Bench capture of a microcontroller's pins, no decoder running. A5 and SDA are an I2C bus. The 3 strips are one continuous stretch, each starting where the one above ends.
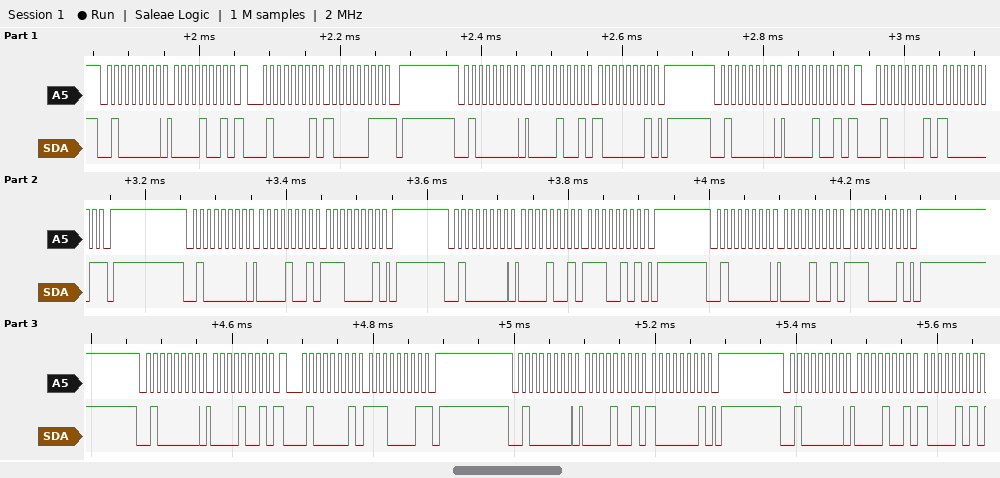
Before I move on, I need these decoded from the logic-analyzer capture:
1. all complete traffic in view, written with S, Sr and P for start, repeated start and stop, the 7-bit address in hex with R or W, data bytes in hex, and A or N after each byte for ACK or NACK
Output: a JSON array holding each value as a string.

["S 20W A 09 A Sr 20R A 83 N P S 20W A 09 A 81 A P S 20W A 09 A Sr 20R A 81 N P S 20W A 09 A E1 A P S 20W A 09 A E5 A P S 20W A 09 A E1 A P S 20W A 09 A Sr 20R A E1 N P S 20W A 09 A 81 A P S 20W A 09 A 85 A"]
